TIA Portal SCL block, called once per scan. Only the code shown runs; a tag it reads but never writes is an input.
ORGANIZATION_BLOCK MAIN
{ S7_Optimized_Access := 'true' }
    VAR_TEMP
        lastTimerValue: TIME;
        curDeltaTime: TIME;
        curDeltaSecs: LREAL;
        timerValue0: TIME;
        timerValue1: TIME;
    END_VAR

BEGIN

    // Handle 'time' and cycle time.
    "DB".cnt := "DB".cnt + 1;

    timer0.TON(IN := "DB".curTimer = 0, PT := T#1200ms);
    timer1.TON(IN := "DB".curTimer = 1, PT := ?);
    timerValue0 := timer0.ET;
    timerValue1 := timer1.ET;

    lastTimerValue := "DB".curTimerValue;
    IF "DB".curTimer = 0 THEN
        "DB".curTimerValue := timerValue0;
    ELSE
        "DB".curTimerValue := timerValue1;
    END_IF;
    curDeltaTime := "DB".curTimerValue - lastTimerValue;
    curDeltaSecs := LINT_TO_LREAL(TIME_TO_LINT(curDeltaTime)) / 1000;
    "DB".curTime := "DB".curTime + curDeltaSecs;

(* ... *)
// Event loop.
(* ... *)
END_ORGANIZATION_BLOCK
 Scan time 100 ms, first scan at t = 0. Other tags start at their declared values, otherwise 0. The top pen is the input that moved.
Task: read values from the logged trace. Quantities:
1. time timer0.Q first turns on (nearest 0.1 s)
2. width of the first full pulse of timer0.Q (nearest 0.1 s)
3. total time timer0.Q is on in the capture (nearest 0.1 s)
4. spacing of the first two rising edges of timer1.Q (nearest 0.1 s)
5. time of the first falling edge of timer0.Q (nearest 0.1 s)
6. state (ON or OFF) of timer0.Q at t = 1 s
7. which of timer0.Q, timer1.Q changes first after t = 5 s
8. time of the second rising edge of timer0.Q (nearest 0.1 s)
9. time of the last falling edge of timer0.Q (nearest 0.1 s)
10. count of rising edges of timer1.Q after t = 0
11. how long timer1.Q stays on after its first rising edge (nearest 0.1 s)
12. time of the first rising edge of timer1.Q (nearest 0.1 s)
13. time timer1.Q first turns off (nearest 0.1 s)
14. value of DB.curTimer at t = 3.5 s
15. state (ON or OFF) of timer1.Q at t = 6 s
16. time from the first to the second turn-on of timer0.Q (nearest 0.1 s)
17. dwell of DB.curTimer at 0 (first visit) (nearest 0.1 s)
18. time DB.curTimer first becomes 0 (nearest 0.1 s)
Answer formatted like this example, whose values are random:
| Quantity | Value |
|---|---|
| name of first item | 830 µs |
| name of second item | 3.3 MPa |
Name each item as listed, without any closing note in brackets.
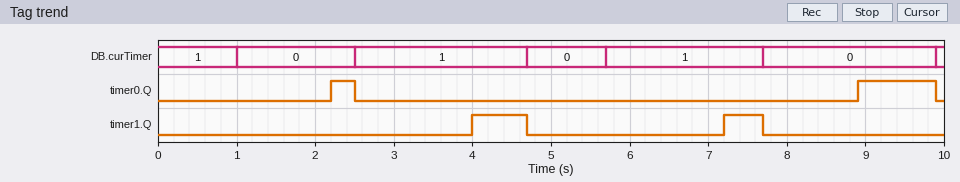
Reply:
| Quantity | Value |
|---|---|
| time timer0.Q first turns on | 2.2 s |
| width of the first full pulse of timer0.Q | 0.3 s |
| total time timer0.Q is on in the capture | 1.3 s |
| spacing of the first two rising edges of timer1.Q | 3.2 s |
| time of the first falling edge of timer0.Q | 2.5 s |
| state (ON or OFF) of timer0.Q at t = 1 s | OFF |
| which of timer0.Q, timer1.Q changes first after t = 5 s | timer1.Q |
| time of the second rising edge of timer0.Q | 8.9 s |
| time of the last falling edge of timer0.Q | 9.9 s |
| count of rising edges of timer1.Q after t = 0 | 2 |
| how long timer1.Q stays on after its first rising edge | 0.7 s |
| time of the first rising edge of timer1.Q | 4.0 s |
| time timer1.Q first turns off | 4.7 s |
| value of DB.curTimer at t = 3.5 s | 1 |
| state (ON or OFF) of timer1.Q at t = 6 s | OFF |
| time from the first to the second turn-on of timer0.Q | 6.7 s |
| dwell of DB.curTimer at 0 (first visit) | 1.5 s |
| time DB.curTimer first becomes 0 | 1.0 s |
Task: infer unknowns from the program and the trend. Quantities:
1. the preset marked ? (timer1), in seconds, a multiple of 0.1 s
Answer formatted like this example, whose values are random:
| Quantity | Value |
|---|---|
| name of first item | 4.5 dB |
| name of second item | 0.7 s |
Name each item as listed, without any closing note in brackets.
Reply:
| Quantity | Value |
|---|---|
| the preset marked ? (timer1), in seconds, a multiple of 0.1 s | 1.5 s |
